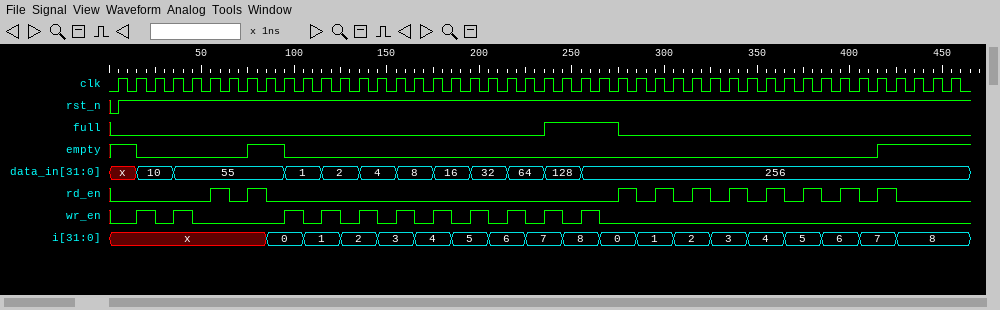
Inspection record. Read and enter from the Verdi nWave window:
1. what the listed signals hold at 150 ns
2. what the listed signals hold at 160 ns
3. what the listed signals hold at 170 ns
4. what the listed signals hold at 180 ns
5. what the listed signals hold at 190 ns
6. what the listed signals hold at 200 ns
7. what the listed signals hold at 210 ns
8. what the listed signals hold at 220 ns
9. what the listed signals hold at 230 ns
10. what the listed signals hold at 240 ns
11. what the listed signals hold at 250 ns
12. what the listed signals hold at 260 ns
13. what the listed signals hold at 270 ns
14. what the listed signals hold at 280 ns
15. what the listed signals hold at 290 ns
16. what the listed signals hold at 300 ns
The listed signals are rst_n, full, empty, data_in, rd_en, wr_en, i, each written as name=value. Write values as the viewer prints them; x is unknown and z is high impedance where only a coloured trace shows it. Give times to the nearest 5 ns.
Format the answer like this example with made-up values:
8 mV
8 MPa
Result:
rst_n=1, full=0, empty=0, data_in=4, rd_en=0, wr_en=0, i=3
rst_n=1, full=0, empty=0, data_in=8, rd_en=0, wr_en=1, i=3
rst_n=1, full=0, empty=0, data_in=8, rd_en=0, wr_en=0, i=4
rst_n=1, full=0, empty=0, data_in=16, rd_en=0, wr_en=1, i=4
rst_n=1, full=0, empty=0, data_in=16, rd_en=0, wr_en=0, i=5
rst_n=1, full=0, empty=0, data_in=32, rd_en=0, wr_en=1, i=5
rst_n=1, full=0, empty=0, data_in=32, rd_en=0, wr_en=0, i=6
rst_n=1, full=0, empty=0, data_in=64, rd_en=0, wr_en=1, i=6
rst_n=1, full=0, empty=0, data_in=64, rd_en=0, wr_en=0, i=7
rst_n=1, full=1, empty=0, data_in=128, rd_en=0, wr_en=1, i=7
rst_n=1, full=1, empty=0, data_in=128, rd_en=0, wr_en=0, i=8
rst_n=1, full=1, empty=0, data_in=256, rd_en=0, wr_en=1, i=8
rst_n=1, full=1, empty=0, data_in=256, rd_en=0, wr_en=0, i=0
rst_n=1, full=0, empty=0, data_in=256, rd_en=1, wr_en=0, i=0
rst_n=1, full=0, empty=0, data_in=256, rd_en=0, wr_en=0, i=1
rst_n=1, full=0, empty=0, data_in=256, rd_en=1, wr_en=0, i=1
